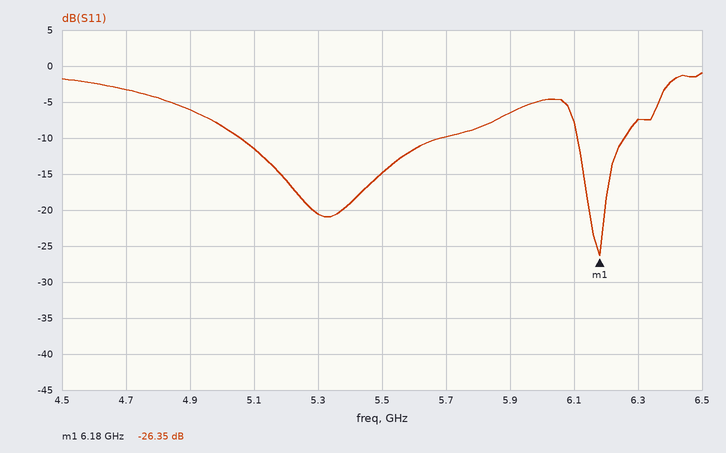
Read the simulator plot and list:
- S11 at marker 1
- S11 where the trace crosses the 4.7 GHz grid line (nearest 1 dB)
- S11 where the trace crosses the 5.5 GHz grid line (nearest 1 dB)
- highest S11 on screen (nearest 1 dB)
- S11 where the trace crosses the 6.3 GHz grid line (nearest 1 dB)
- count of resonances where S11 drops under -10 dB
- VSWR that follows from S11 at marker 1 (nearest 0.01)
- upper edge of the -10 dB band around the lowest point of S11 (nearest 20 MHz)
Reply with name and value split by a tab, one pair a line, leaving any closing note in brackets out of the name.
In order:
S11 at marker 1	-26.35 dB
S11 where the trace crosses the 4.7 GHz grid line	-3 dB
S11 where the trace crosses the 5.5 GHz grid line	-15 dB
highest S11 on screen	-1 dB
S11 where the trace crosses the 6.3 GHz grid line	-7 dB
count of resonances where S11 drops under -10 dB	2
VSWR that follows from S11 at marker 1	1.10
upper edge of the -10 dB band around the lowest point of S11	6.26 GHz
